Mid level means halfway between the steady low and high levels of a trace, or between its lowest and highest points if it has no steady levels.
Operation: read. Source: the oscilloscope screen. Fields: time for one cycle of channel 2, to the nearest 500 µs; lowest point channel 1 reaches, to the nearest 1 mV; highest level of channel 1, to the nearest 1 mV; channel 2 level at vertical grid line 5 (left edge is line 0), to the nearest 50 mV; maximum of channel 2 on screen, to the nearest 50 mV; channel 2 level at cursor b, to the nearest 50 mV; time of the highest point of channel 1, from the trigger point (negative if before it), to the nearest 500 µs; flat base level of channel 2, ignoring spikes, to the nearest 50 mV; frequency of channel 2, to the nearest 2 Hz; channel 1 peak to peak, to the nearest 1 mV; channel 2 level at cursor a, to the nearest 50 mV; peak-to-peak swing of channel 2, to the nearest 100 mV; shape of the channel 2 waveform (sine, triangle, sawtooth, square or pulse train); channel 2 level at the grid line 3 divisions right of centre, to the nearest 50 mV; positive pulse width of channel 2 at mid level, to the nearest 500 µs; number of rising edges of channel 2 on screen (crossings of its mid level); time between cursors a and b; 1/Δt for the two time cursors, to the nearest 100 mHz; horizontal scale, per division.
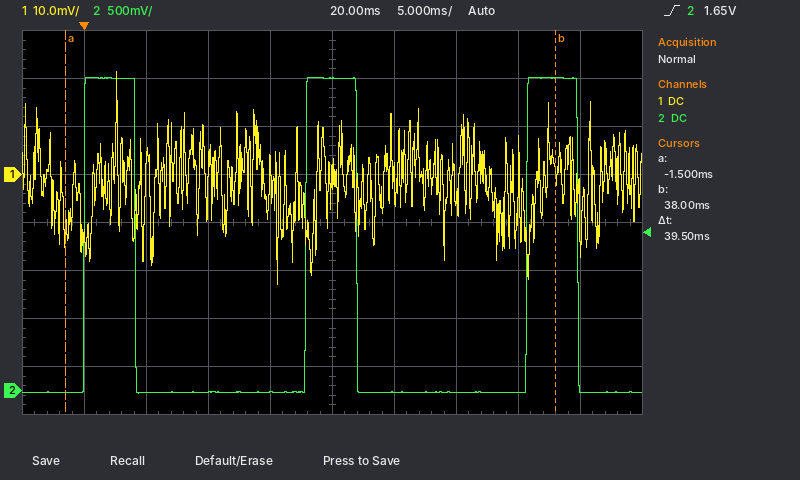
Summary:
18.0 ms
-23 mV
21 mV
3.25 V
3.25 V
3.25 V
+2.5 ms
0 mV
56 Hz
44 mV
0 mV
3.30 V
pulse train
0 mV
4.0 ms
3
39.5 ms
25.3 Hz
5 ms
